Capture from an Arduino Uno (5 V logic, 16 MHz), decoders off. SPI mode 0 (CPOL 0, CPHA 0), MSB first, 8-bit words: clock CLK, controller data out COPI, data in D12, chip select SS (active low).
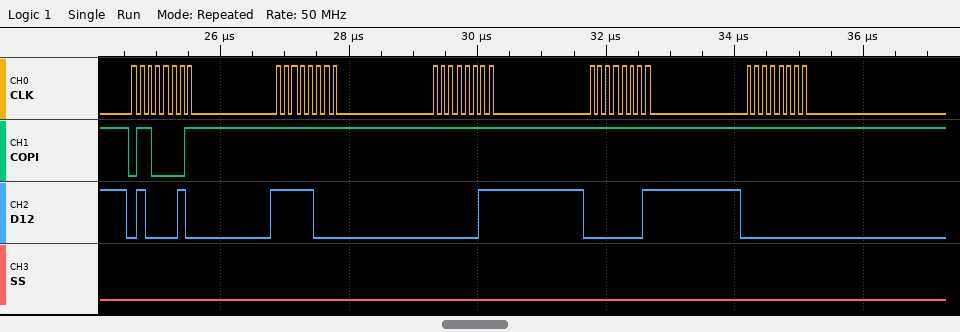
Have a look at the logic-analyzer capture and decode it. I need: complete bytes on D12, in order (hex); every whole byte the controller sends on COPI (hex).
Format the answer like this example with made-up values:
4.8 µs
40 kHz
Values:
42 F8 03 01 00
61 FF FF FF FF
